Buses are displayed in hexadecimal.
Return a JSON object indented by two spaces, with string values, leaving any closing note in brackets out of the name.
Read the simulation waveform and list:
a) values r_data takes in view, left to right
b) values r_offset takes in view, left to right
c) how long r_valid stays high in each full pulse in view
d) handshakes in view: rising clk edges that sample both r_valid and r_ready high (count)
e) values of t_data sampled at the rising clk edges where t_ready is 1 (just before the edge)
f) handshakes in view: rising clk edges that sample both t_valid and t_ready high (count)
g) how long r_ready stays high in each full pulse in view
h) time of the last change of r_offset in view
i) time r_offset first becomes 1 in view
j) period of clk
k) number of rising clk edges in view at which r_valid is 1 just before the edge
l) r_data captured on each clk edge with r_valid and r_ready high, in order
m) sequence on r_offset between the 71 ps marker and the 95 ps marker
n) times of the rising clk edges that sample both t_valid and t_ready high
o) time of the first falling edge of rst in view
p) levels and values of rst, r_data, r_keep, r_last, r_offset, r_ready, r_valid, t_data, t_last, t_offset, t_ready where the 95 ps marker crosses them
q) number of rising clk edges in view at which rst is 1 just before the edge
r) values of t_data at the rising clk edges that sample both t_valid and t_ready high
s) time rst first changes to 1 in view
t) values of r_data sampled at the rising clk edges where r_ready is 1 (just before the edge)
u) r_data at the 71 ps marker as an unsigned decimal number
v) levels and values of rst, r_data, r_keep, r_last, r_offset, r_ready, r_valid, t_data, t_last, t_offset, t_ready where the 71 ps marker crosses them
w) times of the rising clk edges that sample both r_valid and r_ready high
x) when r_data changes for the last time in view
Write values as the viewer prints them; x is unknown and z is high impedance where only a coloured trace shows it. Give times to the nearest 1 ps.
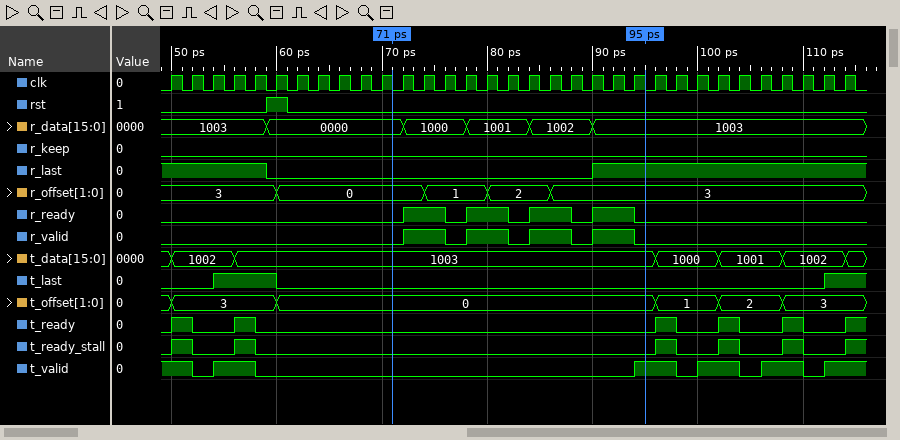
{
  "values r_data takes in view, left to right": "1003, 0000, 1000, 1001, 1002, 1003",
  "values r_offset takes in view, left to right": "3, 0, 1, 2, 3",
  "how long r_valid stays high in each full pulse in view": "4 ps, 4 ps, 4 ps, 4 ps",
  "handshakes in view: rising clk edges that sample both r_valid and r_ready high": "8",
  "values of t_data sampled at the rising clk edges where t_ready is 1": "1002, 1003, 1000, 1001, 1002",
  "handshakes in view: rising clk edges that sample both t_valid and t_ready high": "5",
  "how long r_ready stays high in each full pulse in view": "4 ps, 4 ps, 4 ps, 4 ps",
  "time of the last change of r_offset in view": "86 ps",
  "time r_offset first becomes 1 in view": "74 ps",
  "period of clk": "2 ps",
  "number of rising clk edges in view at which r_valid is 1 just before the edge": "8",
  "r_data captured on each clk edge with r_valid and r_ready high, in order": "1000, 1000, 1001, 1001, 1002, 1002, 1003, 1003",
  "sequence on r_offset between the 71 ps marker and the 95 ps marker": "0, 1, 2, 3",
  "times of the rising clk edges that sample both t_valid and t_ready high": "52 ps, 58 ps, 98 ps, 104 ps, 110 ps",
  "time of the first falling edge of rst in view": "61 ps",
  "levels and values of rst, r_data, r_keep, r_last, r_offset, r_ready, r_valid, t_data, t_last, t_offset, t_ready where the 95 ps marker crosses them": "rst=0, r_data=1003, r_keep=0, r_last=1, r_offset=3, r_ready=0, r_valid=0, t_data=1003, t_last=0, t_offset=0, t_ready=0",
  "number of rising clk edges in view at which rst is 1 just before the edge": "1",
  "values of t_data at the rising clk edges that sample both t_valid and t_ready high": "1002, 1003, 1000, 1001, 1002",
  "time rst first changes to 1 in view": "59 ps",
  "values of r_data sampled at the rising clk edges where r_ready is 1": "1000, 1000, 1001, 1001, 1002, 1002, 1003, 1003",
  "r_data at the 71 ps marker as an unsigned decimal number": "0",
  "levels and values of rst, r_data, r_keep, r_last, r_offset, r_ready, r_valid, t_data, t_last, t_offset, t_ready where the 71 ps marker crosses them": "rst=0, r_data=0000, r_keep=0, r_last=0, r_offset=0, r_ready=0, r_valid=0, t_data=1003, t_last=0, t_offset=0, t_ready=0",
  "times of the rising clk edges that sample both r_valid and r_ready high": "74 ps, 76 ps, 80 ps, 82 ps, 86 ps, 88 ps, 92 ps, 94 ps",
  "when r_data changes for the last time in view": "90 ps"
}
